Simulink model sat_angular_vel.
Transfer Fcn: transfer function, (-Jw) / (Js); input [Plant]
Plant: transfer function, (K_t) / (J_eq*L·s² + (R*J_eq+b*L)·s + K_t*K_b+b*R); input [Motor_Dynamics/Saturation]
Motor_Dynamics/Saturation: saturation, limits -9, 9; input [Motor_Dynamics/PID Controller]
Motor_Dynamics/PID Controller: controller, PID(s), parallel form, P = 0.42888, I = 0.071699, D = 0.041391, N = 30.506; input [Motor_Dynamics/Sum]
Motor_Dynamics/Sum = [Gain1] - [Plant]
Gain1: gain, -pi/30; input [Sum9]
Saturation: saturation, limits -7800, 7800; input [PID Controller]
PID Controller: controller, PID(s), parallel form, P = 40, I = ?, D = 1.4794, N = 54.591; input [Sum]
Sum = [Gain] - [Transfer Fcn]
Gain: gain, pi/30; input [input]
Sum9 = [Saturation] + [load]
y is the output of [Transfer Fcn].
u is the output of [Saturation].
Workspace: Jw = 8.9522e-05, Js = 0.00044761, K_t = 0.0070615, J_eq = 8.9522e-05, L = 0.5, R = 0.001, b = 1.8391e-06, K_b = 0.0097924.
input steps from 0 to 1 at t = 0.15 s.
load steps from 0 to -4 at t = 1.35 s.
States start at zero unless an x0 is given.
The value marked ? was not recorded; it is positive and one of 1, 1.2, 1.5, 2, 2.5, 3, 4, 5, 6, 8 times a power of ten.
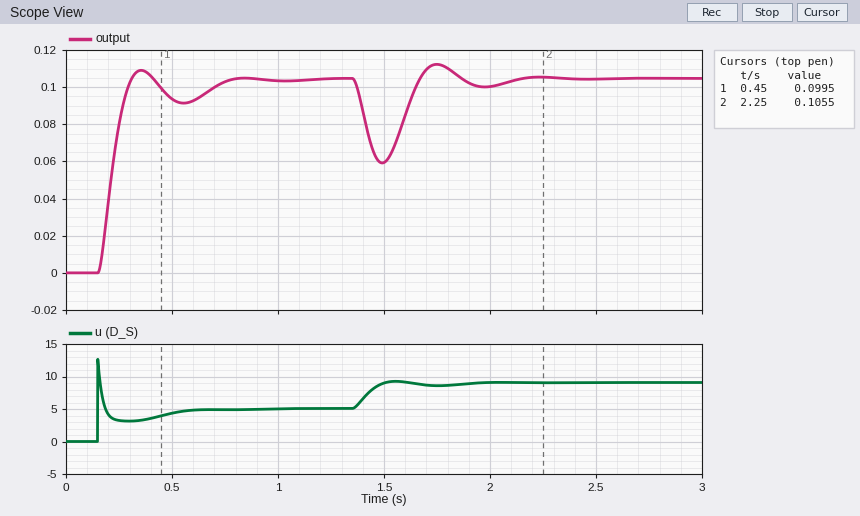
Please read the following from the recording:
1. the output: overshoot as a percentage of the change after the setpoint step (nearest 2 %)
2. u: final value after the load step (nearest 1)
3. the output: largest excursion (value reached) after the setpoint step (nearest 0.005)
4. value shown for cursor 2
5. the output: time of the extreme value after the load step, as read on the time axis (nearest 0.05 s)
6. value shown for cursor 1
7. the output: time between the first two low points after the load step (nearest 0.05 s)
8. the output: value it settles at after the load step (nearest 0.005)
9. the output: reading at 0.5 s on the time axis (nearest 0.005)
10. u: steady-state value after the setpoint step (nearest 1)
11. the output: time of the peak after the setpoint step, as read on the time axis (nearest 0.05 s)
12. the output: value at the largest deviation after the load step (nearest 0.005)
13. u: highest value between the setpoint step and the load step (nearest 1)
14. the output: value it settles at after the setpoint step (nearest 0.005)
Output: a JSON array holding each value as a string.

["4 %", "9", "0.110", "0.1055", "1.50 s", "0.0995", "0.50 s", "0.105", "0.095", "5", "0.35 s", "0.060", "13", "0.105"]
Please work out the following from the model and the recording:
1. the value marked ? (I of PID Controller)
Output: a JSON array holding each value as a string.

["500"]
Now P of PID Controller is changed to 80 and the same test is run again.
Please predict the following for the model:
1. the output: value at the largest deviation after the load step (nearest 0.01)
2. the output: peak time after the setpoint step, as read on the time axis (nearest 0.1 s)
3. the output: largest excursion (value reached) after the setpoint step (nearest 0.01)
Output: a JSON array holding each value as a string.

["0.07", "0.3 s", "0.11"]
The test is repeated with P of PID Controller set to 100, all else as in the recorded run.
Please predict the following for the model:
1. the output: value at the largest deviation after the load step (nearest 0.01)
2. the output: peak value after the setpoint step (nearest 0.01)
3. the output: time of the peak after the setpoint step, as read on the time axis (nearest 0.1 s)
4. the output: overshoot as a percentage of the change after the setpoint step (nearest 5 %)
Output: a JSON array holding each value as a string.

["0.07", "0.11", "0.3 s", "10 %"]
